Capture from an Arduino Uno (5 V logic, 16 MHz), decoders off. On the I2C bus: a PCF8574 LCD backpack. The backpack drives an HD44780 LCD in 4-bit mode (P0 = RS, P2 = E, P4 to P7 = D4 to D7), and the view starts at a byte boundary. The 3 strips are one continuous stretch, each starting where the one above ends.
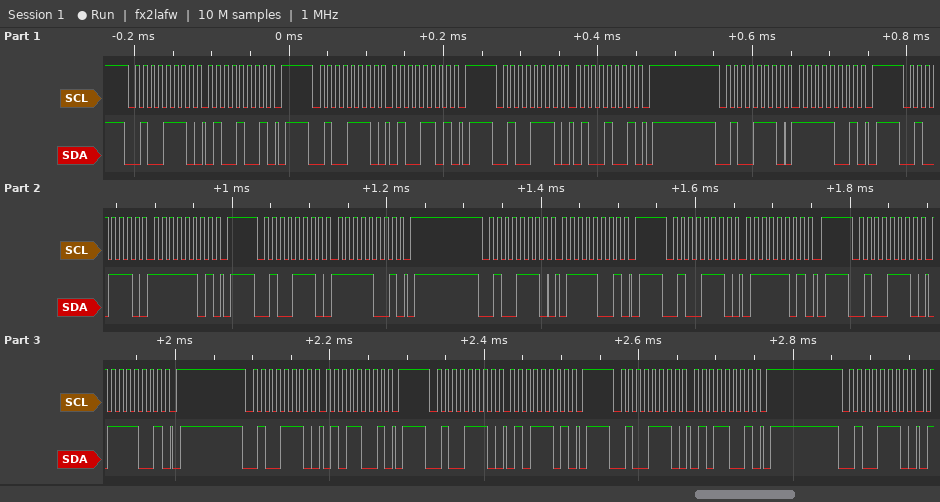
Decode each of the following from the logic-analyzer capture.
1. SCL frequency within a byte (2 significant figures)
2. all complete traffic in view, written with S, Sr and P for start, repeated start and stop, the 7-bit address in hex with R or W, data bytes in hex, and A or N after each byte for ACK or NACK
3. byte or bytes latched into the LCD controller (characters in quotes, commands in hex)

100 kHz
S 27W A 49 A P S 27W A 4D A P S 27W A 49 A P S 27W A F9 A P S 27W A FD A P S 27W A F9 A P S 27W A 79 A P S 27W A 7D A P S 27W A 79 A P S 27W A 59 A P S 27W A 5D A P S 27W A 59 A P S 27W A
'O' 'u'
